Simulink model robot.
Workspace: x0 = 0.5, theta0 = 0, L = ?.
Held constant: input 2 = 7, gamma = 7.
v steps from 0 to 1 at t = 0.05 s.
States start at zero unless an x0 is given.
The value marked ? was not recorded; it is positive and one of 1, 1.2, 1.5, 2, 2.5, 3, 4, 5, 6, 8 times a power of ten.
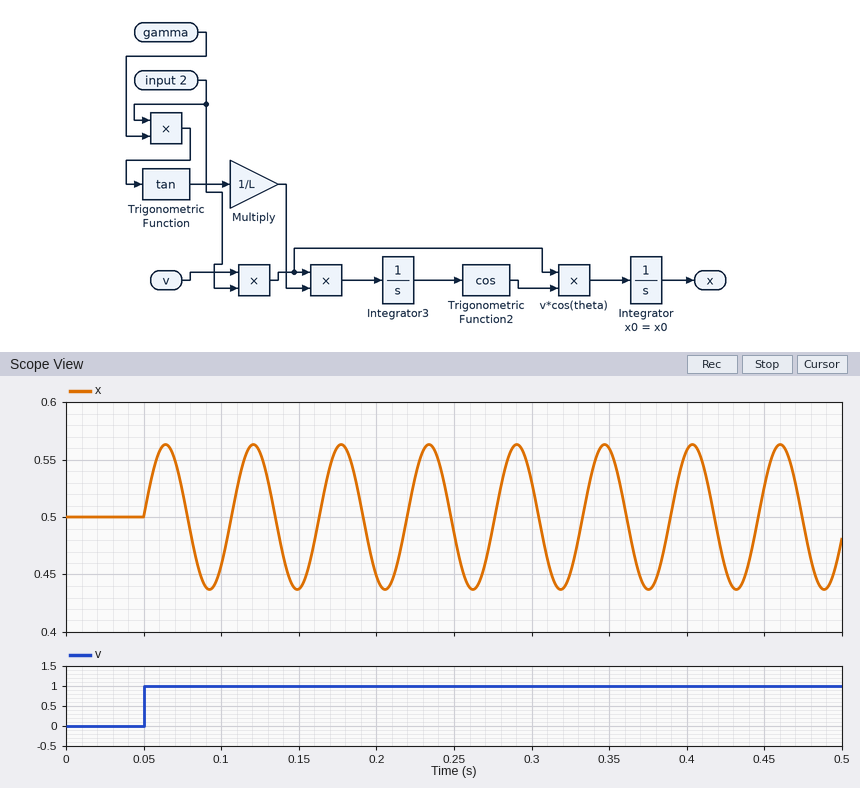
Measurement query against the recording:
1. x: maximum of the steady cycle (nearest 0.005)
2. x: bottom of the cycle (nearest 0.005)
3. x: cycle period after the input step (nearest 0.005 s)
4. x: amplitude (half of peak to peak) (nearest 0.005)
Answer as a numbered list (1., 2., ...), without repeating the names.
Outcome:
1. 0.565
2. 0.435
3. 0.055 s
4. 0.065
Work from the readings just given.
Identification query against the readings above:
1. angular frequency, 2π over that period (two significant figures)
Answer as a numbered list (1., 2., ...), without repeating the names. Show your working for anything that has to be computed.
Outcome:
1. 2π / 0.055 = 110 rad/s
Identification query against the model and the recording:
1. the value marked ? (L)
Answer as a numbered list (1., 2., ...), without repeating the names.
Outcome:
1. 0.2
